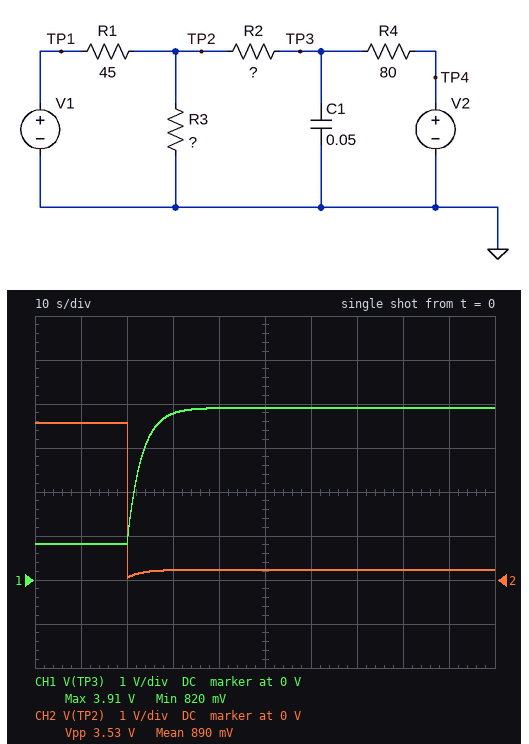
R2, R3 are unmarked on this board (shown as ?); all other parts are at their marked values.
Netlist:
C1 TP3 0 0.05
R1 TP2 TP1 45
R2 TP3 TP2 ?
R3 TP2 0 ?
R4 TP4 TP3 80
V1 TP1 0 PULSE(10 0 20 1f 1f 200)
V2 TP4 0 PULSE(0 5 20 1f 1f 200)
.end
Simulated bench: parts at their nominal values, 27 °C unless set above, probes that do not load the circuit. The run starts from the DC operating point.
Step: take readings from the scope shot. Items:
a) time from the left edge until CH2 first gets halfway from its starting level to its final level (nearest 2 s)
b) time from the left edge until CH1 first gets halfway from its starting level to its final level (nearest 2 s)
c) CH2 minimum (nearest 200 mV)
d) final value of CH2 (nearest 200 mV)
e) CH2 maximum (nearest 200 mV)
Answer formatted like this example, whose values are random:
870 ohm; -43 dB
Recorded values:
20 s; 22 s; 0 V; 200 mV; 3.6 V
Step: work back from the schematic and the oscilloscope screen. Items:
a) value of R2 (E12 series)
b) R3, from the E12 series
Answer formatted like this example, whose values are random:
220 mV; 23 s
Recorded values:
270 Ω; 27 Ω
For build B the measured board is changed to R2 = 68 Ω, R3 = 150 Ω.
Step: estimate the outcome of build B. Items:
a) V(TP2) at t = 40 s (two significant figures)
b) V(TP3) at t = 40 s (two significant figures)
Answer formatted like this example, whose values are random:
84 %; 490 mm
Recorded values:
950 mV; 2.8 V
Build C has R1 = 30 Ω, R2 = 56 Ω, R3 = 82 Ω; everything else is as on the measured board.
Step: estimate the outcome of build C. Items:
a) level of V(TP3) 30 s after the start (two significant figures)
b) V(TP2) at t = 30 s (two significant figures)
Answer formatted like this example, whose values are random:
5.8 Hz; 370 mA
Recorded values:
2.5 V; 700 mV
